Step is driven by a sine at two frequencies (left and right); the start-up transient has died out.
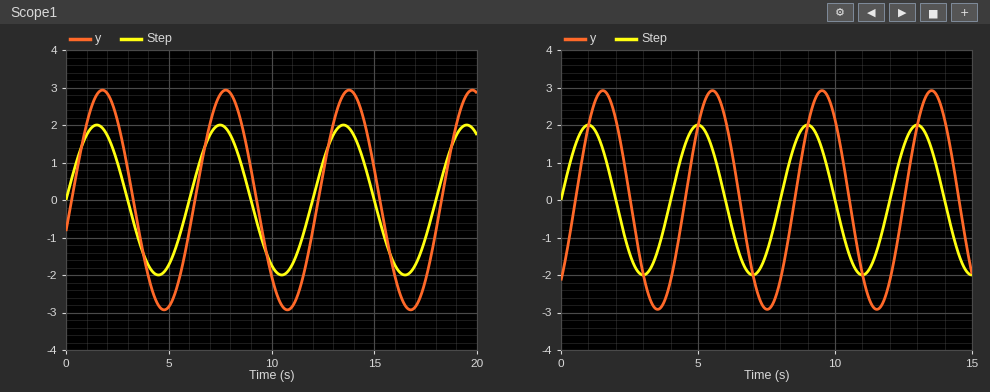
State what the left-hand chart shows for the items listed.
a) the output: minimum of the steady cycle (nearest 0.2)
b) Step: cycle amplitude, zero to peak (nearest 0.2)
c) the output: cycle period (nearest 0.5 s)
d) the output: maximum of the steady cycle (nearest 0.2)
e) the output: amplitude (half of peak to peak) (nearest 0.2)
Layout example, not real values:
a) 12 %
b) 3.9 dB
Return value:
a) -3.0
b) 2.0
c) 6.0 s
d) 3.0
e) 3.0
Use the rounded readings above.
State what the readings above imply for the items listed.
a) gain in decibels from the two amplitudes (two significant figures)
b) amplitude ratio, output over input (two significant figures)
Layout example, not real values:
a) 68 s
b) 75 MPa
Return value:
a) 3.5 dB
b) 1.5
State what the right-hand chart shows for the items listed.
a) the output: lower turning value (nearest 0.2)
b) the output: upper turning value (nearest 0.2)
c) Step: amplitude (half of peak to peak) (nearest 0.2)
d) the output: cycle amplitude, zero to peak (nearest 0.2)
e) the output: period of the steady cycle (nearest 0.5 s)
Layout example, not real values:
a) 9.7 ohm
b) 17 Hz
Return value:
a) -3.0
b) 3.0
c) 2.0
d) 3.0
e) 4.0 s
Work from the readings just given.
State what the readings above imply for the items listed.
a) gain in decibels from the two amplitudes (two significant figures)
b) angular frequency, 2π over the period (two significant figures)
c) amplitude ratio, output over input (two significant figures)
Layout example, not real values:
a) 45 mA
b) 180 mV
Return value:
a) 3.5 dB
b) 1.6 rad/s
c) 1.5
